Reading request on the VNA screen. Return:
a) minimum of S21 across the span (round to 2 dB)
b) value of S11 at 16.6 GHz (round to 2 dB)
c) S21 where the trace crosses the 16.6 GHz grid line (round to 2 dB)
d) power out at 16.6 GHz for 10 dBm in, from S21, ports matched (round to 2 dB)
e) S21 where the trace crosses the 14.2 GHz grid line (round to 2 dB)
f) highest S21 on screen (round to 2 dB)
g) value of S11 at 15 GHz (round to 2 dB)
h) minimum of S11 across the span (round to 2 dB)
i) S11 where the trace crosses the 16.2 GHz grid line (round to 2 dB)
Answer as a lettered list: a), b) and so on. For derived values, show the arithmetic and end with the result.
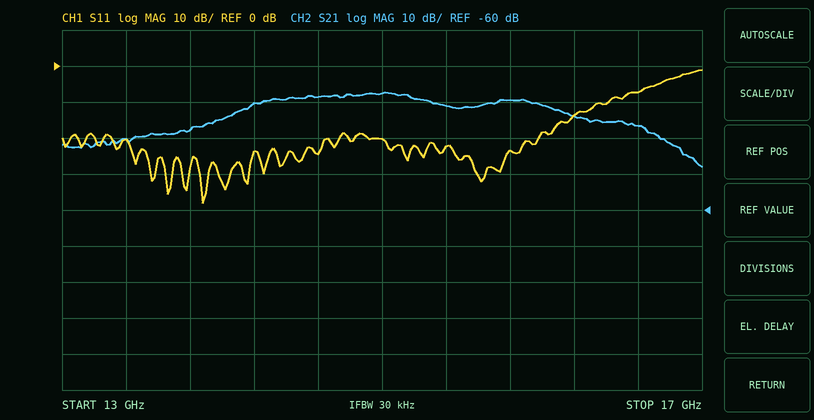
a) -48 dB
b) -8 dB
c) -36 dB
d) 10 dBm + (-36 dB) = -26 dBm
e) -30 dB
f) -28 dB
g) -20 dB
h) -38 dB
i) -14 dB
